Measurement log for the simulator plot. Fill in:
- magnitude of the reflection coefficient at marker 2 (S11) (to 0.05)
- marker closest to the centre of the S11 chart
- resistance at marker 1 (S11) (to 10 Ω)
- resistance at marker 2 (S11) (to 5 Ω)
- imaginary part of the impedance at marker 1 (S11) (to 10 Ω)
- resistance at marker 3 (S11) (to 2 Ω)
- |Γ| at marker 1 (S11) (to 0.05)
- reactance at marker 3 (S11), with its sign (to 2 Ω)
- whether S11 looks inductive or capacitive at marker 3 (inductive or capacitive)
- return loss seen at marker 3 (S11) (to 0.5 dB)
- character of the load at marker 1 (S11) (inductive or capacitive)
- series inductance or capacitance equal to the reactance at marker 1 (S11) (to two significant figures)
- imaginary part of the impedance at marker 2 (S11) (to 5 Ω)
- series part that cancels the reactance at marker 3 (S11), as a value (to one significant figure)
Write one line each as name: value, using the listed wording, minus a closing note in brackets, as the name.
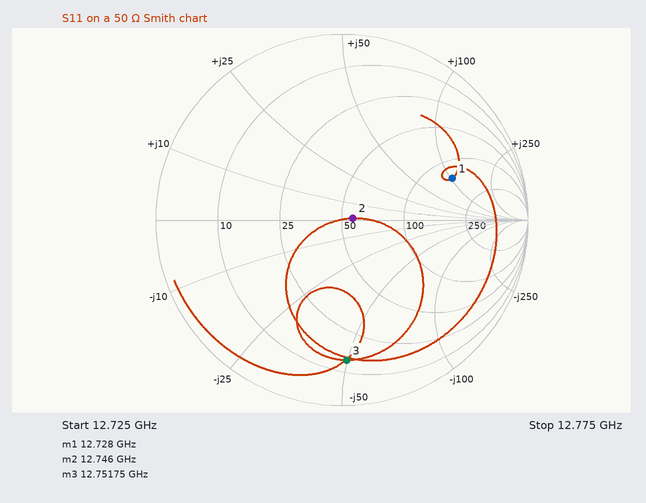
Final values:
magnitude of the reflection coefficient at marker 2 (S11): 0.05
marker closest to the centre of the S11 chart: marker 2
resistance at marker 1 (S11): 140 Ω
resistance at marker 2 (S11): 55 Ω
imaginary part of the impedance at marker 1 (S11): +100 Ω
resistance at marker 3 (S11): 14 Ω
|Γ| at marker 1 (S11): 0.65
reactance at marker 3 (S11), with its sign: -50 Ω
whether S11 looks inductive or capacitive at marker 3: capacitive
return loss seen at marker 3 (S11): 2.5 dB
character of the load at marker 1 (S11): inductive
series inductance or capacitance equal to the reactance at marker 1 (S11): 1.3 nH
imaginary part of the impedance at marker 2 (S11): 0 Ω
series part that cancels the reactance at marker 3 (S11), as a value: 600 pH
